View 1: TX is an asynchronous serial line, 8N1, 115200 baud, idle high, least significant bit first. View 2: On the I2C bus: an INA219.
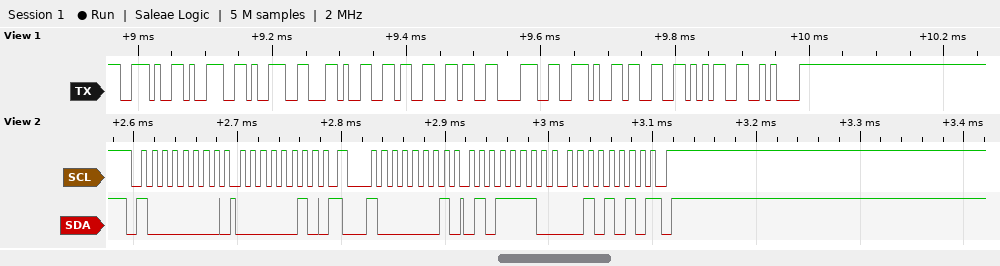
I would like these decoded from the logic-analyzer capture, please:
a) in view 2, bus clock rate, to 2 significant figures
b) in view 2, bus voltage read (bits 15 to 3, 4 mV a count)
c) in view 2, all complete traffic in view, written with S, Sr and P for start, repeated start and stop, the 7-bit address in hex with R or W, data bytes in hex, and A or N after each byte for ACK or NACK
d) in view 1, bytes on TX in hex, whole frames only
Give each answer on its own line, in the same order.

100 kHz
12.052 V
S 40W A 02 A Sr 40R A 5E A 2A N P
2E 39 39 2C 36 36 38 2E 33 35 0A
